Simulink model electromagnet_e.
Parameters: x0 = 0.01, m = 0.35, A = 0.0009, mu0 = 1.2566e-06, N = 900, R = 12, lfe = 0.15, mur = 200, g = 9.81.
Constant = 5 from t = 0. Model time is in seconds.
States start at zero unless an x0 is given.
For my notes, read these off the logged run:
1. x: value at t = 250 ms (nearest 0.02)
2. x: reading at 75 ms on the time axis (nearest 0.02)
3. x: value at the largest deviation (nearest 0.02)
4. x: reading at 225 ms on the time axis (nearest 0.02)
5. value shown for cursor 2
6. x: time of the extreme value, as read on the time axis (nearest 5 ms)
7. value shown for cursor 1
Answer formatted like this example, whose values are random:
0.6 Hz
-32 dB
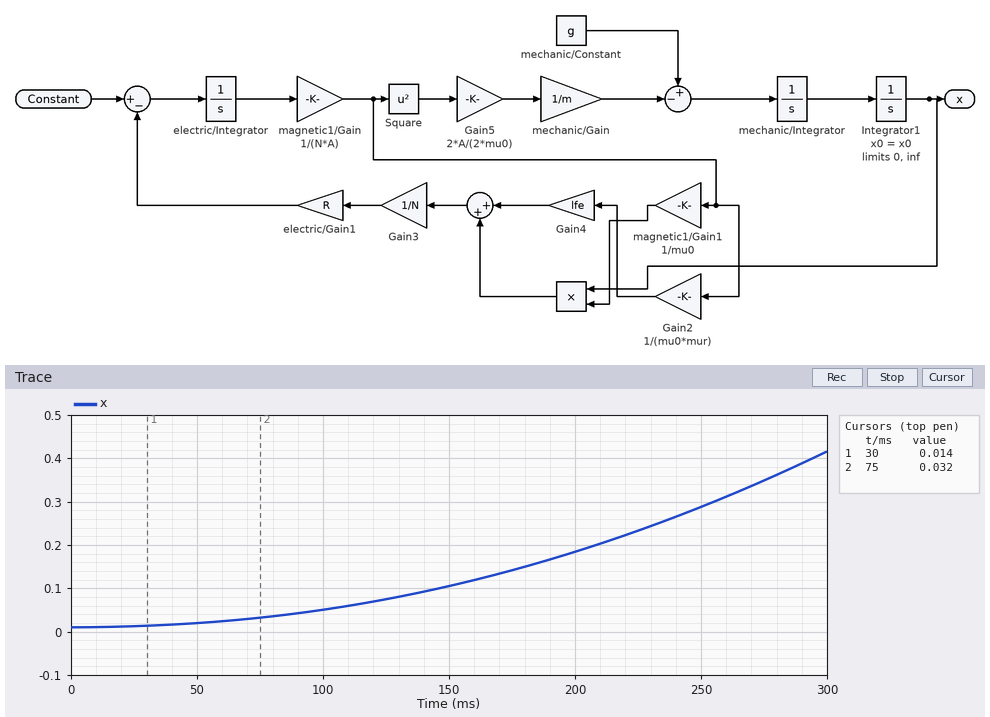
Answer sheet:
0.28
0.04
0.42
0.24
0.032
300 ms
0.014
